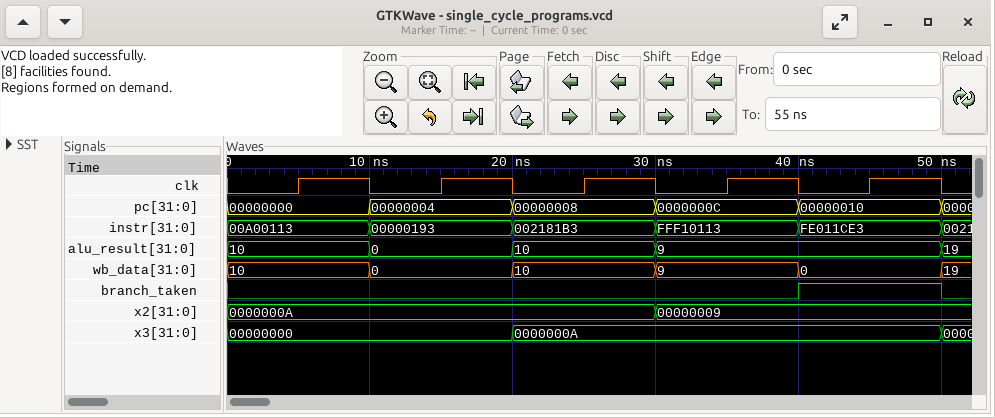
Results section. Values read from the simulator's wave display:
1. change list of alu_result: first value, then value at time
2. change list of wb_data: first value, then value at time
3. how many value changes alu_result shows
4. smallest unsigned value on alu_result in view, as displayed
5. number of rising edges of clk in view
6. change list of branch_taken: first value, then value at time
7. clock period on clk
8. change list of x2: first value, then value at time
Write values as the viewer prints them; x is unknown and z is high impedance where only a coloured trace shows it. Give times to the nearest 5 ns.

10, 0 at 10 ns, 10 at 20 ns, 9 at 30 ns, 19 at 50 ns
10, 0 at 10 ns, 10 at 20 ns, 9 at 30 ns, 0 at 40 ns, 19 at 50 ns
4
0
5
0, 1 at 40 ns, 0 at 50 ns
10 ns
0000000A, 00000009 at 30 ns
